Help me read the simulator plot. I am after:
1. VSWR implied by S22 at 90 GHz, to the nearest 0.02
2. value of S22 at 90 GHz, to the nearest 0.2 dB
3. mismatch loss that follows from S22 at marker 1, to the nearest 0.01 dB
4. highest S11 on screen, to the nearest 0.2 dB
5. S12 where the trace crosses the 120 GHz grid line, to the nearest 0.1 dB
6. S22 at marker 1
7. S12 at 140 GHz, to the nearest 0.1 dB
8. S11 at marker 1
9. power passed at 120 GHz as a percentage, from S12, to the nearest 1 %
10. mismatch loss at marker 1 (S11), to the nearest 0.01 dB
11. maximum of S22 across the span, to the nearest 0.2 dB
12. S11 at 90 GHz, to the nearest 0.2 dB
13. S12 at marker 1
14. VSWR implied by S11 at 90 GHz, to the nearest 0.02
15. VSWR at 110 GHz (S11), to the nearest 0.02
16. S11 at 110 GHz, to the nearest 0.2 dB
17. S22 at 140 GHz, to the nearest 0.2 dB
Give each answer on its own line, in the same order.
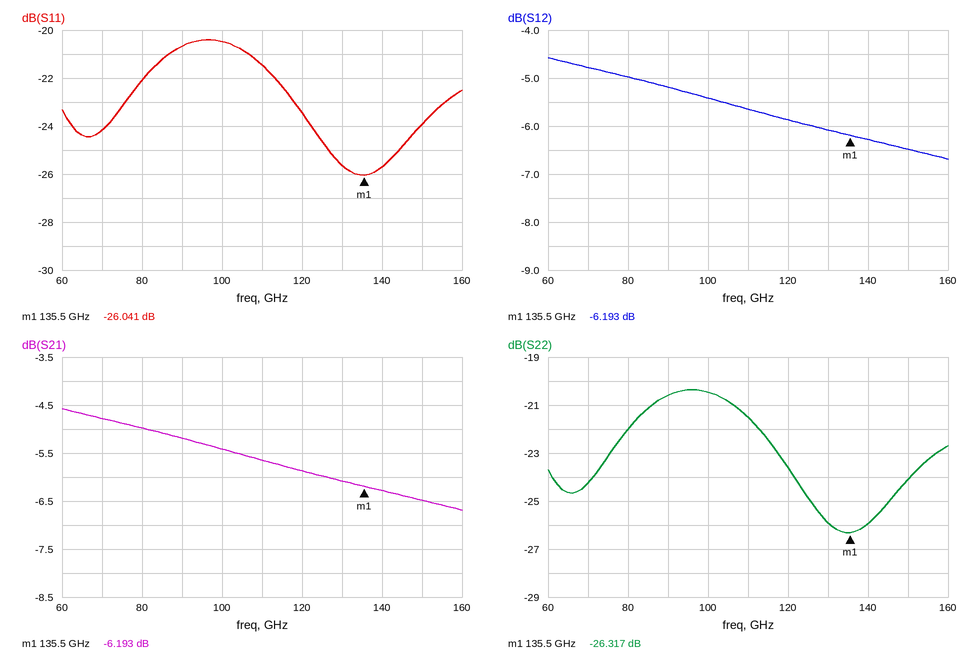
1.20
-20.6 dB
0.01 dB
-20.4 dB
-5.9 dB
-26.317 dB
-6.3 dB
-26.041 dB
26 %
0.01 dB
-20.4 dB
-20.6 dB
-6.193 dB
1.20
1.18
-21.4 dB
-26.0 dB
